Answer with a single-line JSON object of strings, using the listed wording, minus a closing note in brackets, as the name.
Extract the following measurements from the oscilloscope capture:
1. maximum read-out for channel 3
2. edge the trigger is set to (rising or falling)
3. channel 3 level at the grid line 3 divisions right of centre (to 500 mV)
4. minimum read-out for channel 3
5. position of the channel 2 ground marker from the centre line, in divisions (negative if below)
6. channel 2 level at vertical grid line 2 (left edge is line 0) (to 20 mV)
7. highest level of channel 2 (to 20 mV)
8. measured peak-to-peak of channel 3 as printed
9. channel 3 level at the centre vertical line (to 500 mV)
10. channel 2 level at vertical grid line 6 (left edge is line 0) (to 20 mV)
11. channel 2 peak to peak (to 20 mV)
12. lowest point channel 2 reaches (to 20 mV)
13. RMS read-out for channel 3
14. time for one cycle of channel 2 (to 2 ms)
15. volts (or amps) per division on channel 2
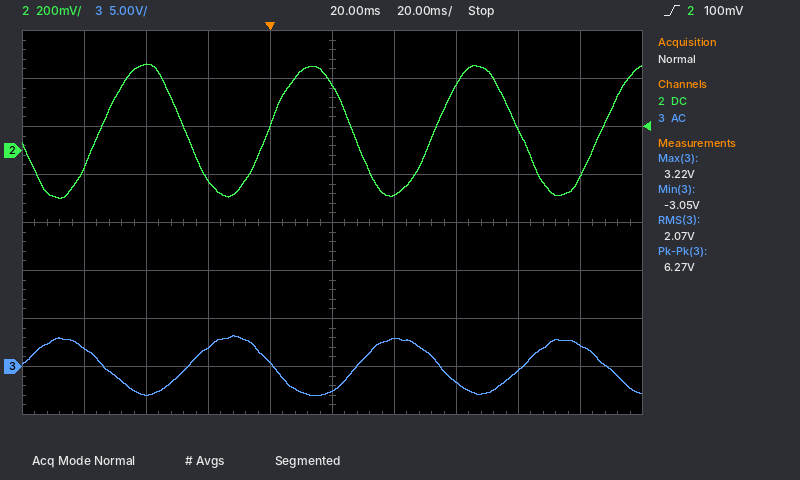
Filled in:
{"maximum read-out for channel 3": "3.22 V", "edge the trigger is set to": "rising", "channel 3 level at the grid line 3 divisions right of centre": "-500 mV", "minimum read-out for channel 3": "-3.05 V", "position of the channel 2 ground marker from the centre line, in divisions": "+1.5 div", "channel 2 level at vertical grid line 2 (left edge is line 0)": "360 mV", "highest level of channel 2": "360 mV", "measured peak-to-peak of channel 3 as printed": "6.27 V", "channel 3 level at the centre vertical line": "-2.5 V", "channel 2 level at vertical grid line 6 (left edge is line 0)": "-180 mV", "channel 2 peak to peak": "560 mV", "lowest point channel 2 reaches": "-200 mV", "RMS read-out for channel 3": "2.07 V", "time for one cycle of channel 2": "54 ms", "volts (or amps) per division on channel 2": "200 mV"}
